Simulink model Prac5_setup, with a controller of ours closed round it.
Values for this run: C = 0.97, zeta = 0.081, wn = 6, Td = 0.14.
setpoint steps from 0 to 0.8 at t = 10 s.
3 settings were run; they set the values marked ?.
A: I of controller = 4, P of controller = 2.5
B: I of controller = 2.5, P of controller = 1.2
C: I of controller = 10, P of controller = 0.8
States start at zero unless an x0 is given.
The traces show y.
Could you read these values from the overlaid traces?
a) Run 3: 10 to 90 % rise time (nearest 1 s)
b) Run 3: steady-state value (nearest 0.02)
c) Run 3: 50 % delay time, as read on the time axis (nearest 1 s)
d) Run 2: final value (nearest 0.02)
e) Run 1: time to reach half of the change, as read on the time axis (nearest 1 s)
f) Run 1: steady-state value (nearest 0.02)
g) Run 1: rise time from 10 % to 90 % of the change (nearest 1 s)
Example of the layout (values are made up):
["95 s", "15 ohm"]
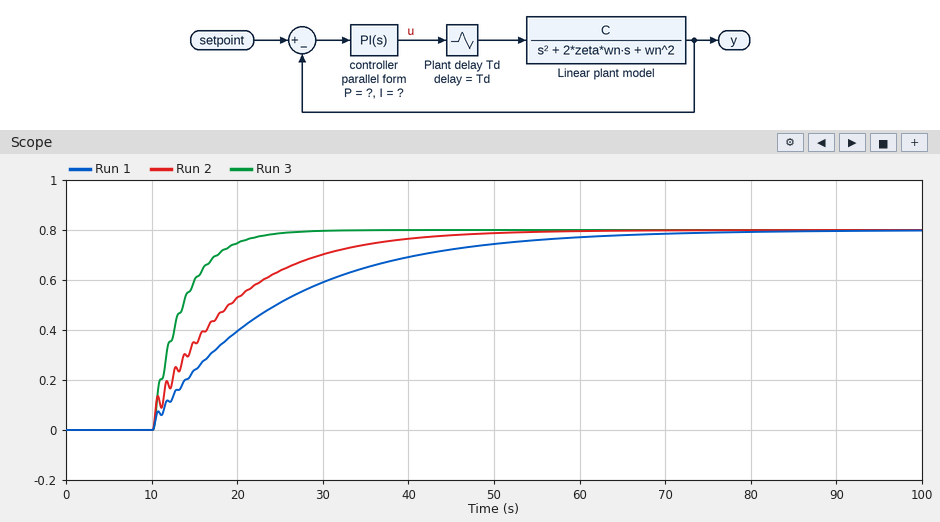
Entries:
["8 s", "0.80", "13 s", "0.80", "20 s", "0.80", "33 s"]
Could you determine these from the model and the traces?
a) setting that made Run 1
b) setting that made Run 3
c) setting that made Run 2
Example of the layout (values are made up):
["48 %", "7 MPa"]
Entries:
["B", "C", "A"]
